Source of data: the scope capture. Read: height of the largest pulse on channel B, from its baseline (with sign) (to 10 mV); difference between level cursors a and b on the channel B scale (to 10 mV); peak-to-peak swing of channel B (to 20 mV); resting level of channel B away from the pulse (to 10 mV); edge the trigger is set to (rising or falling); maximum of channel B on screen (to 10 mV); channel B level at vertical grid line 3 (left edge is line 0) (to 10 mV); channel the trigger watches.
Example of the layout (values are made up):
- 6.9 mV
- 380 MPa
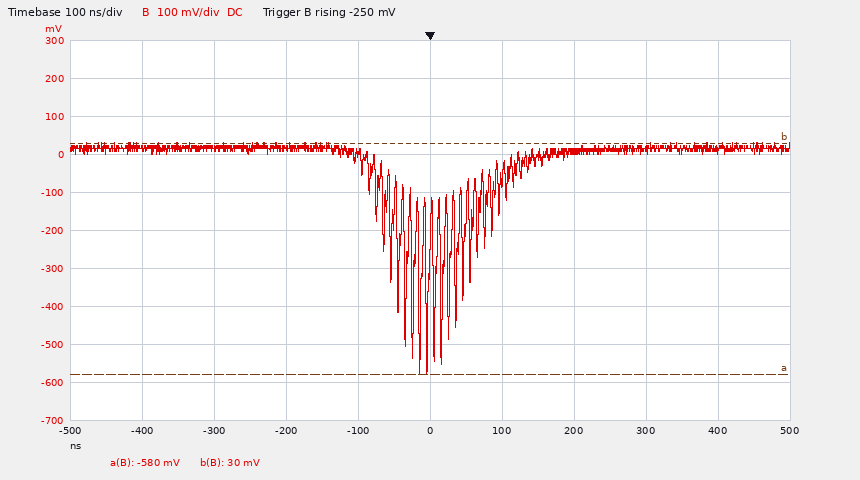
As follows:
- -590 mV
- 610 mV
- 600 mV
- 20 mV
- rising
- 30 mV
- 20 mV
- channel B
